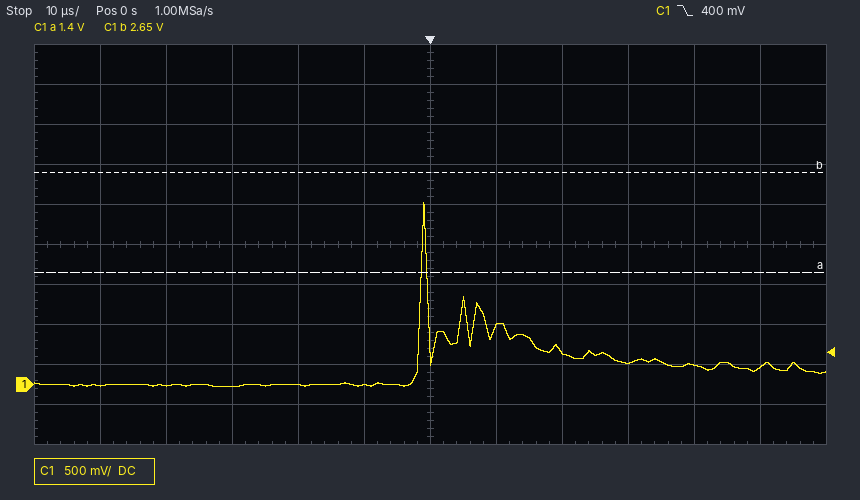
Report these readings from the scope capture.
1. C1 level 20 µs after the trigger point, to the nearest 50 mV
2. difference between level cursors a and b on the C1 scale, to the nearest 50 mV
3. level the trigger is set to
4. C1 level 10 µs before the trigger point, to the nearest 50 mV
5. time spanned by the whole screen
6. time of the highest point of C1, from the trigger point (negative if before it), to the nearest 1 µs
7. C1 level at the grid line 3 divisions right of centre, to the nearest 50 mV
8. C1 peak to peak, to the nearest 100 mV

400 mV
1.25 V
400 mV
0 mV
120 µs
-1 µs
250 mV
2.30 V
